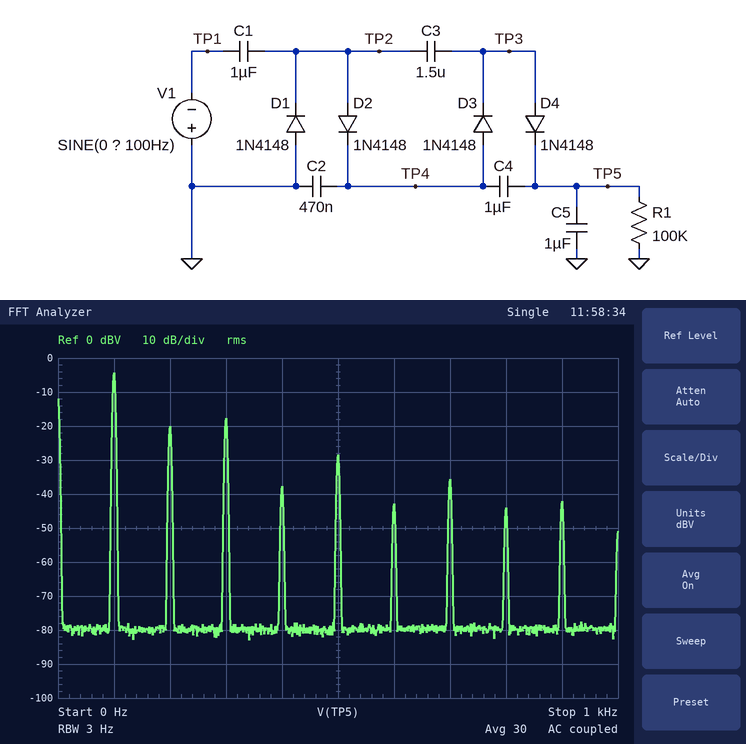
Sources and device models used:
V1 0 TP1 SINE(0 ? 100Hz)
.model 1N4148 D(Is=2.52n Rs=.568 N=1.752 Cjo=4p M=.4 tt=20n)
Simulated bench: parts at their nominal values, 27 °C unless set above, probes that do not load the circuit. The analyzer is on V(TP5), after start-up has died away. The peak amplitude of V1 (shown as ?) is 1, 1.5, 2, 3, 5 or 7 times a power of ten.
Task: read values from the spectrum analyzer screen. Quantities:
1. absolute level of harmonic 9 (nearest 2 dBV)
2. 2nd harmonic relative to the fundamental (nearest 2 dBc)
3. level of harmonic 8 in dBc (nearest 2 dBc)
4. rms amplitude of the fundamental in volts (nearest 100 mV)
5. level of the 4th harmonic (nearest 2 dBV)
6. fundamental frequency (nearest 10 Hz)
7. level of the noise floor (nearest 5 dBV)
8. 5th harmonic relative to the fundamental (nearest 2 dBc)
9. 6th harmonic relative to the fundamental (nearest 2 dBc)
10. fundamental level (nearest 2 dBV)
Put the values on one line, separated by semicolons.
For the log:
-42 dBV; -16 dBc; -40 dBc; 600 mV; -38 dBV; 100 Hz; -80 dBV; -24 dBc; -38 dBc; -4 dBV
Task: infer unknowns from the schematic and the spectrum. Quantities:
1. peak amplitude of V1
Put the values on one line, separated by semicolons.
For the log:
7 V
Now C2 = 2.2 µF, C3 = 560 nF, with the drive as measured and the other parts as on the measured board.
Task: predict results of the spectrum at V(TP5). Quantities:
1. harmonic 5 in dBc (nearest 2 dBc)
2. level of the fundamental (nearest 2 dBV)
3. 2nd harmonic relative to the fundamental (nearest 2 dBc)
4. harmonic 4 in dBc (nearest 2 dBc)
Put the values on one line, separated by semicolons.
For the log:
-26 dBc; -10 dBV; -12 dBc; -30 dBc
